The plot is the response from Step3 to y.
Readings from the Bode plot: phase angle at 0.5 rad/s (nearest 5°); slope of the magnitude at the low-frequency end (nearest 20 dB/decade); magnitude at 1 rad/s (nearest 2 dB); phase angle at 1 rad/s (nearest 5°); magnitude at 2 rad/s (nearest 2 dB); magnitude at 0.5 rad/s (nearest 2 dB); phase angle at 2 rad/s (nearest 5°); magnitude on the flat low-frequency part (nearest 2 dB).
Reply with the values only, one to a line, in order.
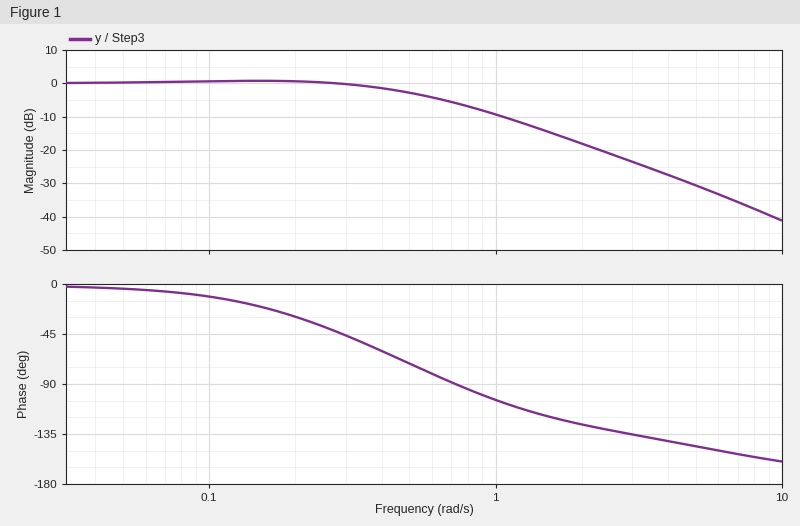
-70°
0 dB/decade
-10 dB
-105°
-18 dB
-2 dB
-125°
0 dB
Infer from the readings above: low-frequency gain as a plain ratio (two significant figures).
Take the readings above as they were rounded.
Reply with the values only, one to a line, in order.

1.0
